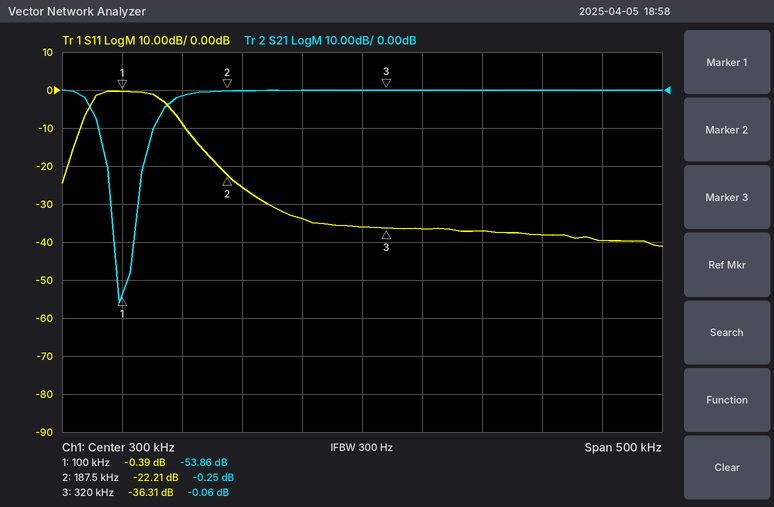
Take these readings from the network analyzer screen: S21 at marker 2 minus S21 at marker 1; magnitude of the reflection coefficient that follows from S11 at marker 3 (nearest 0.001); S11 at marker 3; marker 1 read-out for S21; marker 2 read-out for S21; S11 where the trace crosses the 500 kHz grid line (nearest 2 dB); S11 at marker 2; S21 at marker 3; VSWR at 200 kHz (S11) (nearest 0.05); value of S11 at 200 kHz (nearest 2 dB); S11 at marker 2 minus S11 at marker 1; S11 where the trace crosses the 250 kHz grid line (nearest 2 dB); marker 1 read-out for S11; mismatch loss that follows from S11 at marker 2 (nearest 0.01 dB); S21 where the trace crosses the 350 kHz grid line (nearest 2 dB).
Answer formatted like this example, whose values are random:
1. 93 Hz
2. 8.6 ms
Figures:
1. 53.61 dB
2. 0.015
3. -36.31 dB
4. -53.86 dB
5. -0.25 dB
6. -40 dB
7. -22.21 dB
8. -0.06 dB
9. 1.10
10. -26 dB
11. -21.82 dB
12. -34 dB
13. -0.39 dB
14. 0.03 dB
15. 0 dB
